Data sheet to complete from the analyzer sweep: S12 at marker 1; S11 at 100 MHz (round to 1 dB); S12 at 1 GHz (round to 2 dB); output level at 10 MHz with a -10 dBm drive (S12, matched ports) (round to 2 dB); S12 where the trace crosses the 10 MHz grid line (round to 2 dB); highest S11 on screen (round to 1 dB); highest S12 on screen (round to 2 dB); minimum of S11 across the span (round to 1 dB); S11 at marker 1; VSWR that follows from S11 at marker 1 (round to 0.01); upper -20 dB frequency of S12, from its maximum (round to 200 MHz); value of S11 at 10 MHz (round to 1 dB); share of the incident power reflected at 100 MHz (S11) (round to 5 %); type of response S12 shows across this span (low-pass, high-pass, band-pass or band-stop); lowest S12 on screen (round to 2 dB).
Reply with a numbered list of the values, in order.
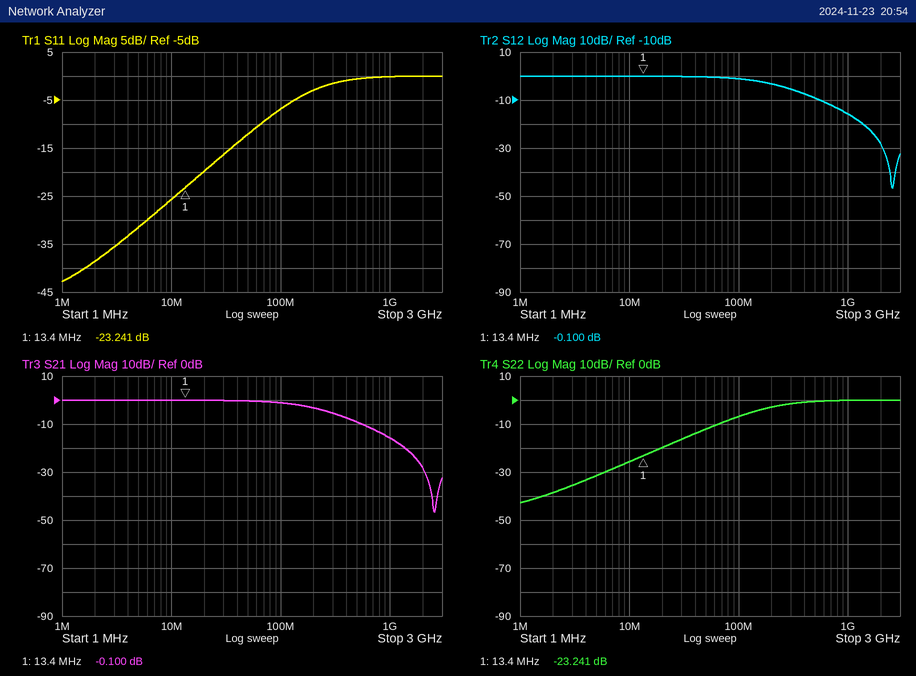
1. -0.100 dB
2. -7 dB
3. -16 dB
4. -10 dBm
5. 0 dB
6. 0 dB
7. 0 dB
8. -43 dB
9. -23.241 dB
10. 1.15
11. 1.4 GHz
12. -26 dB
13. 20 %
14. low-pass
15. -46 dB
